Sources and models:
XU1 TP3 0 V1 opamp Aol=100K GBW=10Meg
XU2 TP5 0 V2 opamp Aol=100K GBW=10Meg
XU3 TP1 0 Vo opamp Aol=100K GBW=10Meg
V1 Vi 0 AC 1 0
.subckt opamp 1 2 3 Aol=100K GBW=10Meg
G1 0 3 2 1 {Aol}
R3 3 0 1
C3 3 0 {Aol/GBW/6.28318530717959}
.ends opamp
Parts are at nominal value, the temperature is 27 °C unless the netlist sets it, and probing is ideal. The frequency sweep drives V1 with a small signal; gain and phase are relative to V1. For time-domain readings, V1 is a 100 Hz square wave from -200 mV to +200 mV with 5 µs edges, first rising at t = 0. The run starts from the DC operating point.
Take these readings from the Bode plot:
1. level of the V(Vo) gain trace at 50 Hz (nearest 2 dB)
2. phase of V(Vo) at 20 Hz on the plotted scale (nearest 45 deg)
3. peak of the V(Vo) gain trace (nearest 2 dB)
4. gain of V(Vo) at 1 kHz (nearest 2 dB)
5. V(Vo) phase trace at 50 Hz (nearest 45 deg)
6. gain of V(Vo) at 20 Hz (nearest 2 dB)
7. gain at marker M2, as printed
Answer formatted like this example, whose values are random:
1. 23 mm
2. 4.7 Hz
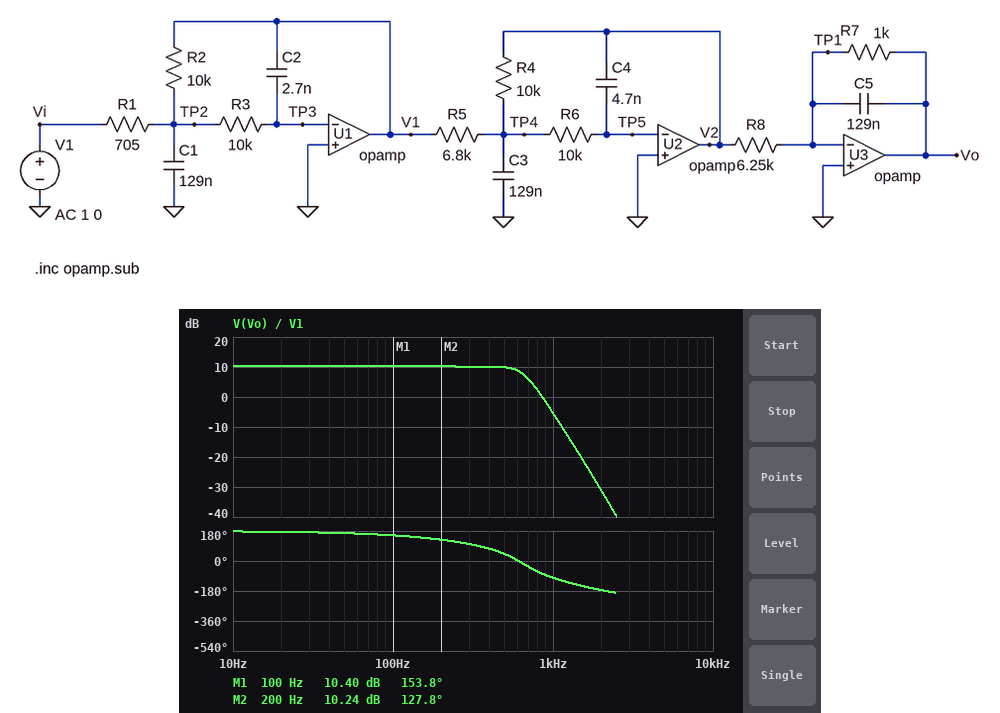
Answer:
1. 10 dB
2. 180 deg
3. 10 dB
4. -6 dB
5. 180 deg
6. 10 dB
7. 10.24 dB
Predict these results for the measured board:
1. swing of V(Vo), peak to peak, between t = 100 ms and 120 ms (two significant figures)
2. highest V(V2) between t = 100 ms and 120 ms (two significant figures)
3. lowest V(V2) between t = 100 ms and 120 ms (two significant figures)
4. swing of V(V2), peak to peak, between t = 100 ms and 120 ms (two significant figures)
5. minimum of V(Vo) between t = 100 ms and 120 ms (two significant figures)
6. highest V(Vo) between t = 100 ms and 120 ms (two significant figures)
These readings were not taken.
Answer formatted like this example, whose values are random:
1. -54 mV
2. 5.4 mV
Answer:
1. 1.6 V
2. 5.1 V
3. -5.1 V
4. 10 V
5. -790 mV
6. 790 mV
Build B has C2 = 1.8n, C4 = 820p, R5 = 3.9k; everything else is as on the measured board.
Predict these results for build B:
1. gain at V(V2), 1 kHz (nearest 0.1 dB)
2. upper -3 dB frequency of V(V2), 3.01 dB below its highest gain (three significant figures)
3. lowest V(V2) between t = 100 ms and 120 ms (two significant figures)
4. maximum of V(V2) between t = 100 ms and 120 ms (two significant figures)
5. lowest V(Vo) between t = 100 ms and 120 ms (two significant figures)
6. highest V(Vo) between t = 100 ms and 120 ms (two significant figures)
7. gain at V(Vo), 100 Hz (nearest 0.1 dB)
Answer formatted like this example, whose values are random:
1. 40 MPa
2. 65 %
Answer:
1. 30.0 dB
2. 1.66 kHz
3. -8.3 V
4. 8.3 V
5. -1.2 V
6. 1.2 V
7. 15.2 dB
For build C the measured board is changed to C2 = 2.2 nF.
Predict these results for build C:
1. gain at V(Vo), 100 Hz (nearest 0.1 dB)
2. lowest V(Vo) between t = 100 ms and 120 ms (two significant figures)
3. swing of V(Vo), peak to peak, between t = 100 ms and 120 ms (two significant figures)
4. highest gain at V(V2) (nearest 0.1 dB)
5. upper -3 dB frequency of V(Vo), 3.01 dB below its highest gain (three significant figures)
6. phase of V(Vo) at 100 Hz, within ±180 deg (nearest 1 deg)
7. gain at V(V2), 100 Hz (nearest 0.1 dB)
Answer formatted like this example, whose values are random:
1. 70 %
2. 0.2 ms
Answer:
1. 10.5 dB
2. -870 mV
3. 1.7 V
4. 27.6 dB
5. 687 Hz
6. 157 deg
7. 26.4 dB
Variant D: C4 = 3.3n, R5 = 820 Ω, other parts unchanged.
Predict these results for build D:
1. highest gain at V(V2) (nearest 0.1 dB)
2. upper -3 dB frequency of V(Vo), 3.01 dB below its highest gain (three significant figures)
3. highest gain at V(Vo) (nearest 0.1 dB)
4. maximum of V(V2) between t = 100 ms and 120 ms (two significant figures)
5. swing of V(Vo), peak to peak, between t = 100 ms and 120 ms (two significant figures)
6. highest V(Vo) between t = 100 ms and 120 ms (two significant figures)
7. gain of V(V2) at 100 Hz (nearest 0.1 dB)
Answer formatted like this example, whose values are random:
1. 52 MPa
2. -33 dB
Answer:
1. 44.8 dB
2. 270 Hz
3. 28.8 dB
4. 35 V
5. 11 V
6. 5.5 V
7. 44.3 dB
